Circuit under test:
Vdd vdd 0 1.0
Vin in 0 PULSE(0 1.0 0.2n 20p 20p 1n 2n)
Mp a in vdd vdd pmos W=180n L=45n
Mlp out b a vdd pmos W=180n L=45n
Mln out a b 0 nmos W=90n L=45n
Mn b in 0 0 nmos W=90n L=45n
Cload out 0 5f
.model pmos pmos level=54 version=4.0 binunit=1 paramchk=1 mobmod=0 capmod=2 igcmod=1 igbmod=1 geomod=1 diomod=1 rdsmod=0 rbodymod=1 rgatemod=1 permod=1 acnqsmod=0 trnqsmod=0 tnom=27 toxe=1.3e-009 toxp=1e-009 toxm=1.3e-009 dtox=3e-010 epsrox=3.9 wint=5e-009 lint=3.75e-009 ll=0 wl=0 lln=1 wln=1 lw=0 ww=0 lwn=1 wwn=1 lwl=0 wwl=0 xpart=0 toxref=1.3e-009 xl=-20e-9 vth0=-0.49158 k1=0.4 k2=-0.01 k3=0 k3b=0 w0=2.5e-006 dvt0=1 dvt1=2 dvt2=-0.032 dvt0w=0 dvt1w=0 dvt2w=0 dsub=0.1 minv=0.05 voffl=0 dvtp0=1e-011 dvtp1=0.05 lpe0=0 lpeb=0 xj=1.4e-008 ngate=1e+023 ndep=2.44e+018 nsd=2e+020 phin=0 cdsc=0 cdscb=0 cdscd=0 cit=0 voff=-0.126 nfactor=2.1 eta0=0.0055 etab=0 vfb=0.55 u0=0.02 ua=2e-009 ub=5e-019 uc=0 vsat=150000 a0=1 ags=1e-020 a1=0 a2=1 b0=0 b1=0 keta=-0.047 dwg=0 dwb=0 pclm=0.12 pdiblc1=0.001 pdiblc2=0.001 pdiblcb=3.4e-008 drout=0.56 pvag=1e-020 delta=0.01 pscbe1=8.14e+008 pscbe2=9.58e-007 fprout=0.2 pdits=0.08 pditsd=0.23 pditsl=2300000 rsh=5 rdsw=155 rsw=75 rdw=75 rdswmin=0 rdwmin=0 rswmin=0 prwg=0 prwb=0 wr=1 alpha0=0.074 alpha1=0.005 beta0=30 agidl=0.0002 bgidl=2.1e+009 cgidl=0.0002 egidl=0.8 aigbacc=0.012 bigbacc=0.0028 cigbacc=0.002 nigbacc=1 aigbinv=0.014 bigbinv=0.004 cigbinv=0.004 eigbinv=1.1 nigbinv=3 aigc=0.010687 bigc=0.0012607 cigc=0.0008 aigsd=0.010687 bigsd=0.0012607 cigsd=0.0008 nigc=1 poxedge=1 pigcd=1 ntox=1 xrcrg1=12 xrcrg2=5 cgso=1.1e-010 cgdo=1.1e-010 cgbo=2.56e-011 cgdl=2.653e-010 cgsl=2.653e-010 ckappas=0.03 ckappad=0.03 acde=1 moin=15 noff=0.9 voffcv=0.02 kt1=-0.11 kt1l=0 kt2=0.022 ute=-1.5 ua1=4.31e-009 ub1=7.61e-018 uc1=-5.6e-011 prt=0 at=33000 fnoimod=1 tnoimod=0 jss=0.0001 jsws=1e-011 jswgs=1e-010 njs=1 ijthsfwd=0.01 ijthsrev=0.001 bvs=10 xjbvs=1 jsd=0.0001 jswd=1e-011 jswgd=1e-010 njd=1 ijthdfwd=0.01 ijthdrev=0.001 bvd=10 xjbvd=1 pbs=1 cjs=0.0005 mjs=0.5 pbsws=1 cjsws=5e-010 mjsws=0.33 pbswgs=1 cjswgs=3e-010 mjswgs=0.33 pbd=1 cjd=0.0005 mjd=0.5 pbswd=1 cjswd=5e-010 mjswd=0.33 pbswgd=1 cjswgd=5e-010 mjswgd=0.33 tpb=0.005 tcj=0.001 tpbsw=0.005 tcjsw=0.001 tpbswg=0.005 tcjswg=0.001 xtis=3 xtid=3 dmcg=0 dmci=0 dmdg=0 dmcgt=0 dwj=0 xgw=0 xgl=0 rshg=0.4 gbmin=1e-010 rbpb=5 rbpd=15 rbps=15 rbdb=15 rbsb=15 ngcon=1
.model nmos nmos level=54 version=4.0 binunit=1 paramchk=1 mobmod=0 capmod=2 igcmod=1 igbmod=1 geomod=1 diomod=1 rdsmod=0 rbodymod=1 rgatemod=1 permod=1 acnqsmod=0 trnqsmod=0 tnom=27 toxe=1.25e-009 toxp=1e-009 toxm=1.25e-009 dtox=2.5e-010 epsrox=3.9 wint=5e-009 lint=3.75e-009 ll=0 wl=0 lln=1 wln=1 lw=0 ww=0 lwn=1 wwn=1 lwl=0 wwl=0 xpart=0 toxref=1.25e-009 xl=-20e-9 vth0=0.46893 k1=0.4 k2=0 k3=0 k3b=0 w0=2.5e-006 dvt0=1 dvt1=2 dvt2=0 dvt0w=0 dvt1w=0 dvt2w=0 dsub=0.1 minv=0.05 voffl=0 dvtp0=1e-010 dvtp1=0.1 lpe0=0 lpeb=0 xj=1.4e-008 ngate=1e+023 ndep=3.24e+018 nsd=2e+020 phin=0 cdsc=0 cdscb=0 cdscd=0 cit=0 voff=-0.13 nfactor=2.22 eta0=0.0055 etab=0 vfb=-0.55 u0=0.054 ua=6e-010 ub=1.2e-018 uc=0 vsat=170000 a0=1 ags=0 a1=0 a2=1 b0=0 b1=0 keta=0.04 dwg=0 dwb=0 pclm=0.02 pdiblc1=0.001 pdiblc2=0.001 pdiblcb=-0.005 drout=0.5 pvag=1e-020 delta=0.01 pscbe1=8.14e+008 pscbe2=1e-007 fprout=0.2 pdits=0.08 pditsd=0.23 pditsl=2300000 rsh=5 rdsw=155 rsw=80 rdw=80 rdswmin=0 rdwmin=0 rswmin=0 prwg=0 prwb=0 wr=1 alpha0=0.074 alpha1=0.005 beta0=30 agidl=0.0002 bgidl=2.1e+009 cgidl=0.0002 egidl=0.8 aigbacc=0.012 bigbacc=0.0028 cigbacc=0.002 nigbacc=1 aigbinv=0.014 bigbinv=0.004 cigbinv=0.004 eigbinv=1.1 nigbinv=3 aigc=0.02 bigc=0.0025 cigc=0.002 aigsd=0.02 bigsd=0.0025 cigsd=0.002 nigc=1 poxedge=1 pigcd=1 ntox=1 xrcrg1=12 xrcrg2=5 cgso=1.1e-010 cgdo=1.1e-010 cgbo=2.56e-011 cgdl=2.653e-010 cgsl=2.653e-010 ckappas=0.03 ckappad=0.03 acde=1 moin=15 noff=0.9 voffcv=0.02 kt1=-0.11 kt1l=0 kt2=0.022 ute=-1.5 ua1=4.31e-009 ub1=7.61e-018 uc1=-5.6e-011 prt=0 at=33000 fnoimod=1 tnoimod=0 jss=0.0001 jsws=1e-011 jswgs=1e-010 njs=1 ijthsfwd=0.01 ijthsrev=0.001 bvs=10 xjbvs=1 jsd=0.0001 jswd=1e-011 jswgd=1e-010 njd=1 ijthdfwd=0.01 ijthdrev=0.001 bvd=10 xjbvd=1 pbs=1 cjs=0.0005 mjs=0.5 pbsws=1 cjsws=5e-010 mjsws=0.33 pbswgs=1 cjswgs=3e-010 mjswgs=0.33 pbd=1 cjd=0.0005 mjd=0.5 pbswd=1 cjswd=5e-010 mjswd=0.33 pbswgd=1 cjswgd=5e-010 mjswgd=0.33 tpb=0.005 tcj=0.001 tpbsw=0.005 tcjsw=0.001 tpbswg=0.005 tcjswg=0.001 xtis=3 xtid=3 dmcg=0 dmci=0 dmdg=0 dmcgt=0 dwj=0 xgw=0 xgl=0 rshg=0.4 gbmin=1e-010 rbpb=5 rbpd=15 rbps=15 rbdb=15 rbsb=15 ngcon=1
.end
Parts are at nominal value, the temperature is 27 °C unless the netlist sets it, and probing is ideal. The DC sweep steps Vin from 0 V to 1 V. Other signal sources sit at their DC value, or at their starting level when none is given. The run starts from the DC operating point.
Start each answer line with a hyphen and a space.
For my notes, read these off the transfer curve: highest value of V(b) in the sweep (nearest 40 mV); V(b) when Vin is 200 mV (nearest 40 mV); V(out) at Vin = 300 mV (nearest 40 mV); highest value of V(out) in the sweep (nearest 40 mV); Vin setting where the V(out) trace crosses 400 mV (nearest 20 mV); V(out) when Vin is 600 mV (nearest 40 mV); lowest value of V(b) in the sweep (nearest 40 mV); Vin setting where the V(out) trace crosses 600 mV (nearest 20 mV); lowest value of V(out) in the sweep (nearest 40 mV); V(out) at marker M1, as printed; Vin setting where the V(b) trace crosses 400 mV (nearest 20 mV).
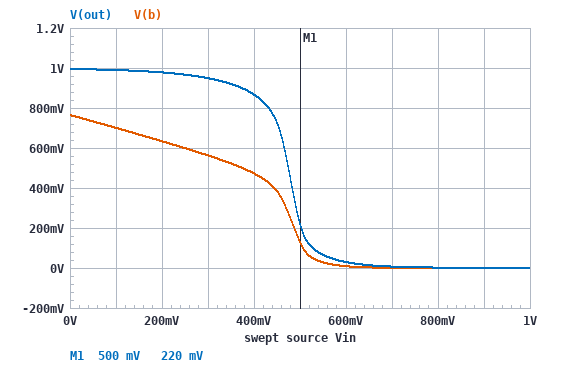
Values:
- 760 mV
- 640 mV
- 960 mV
- 1.00 V
- 480 mV
- 40 mV
- 0 V
- 460 mV
- 0 V
- 220 mV
- 440 mV
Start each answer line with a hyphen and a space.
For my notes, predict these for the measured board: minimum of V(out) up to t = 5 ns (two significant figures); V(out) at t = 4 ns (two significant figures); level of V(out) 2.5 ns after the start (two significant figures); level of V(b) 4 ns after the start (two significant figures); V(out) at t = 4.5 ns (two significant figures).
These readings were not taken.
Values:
- 120 mV
- 680 mV
- 260 mV
- 640 mV
- 260 mV
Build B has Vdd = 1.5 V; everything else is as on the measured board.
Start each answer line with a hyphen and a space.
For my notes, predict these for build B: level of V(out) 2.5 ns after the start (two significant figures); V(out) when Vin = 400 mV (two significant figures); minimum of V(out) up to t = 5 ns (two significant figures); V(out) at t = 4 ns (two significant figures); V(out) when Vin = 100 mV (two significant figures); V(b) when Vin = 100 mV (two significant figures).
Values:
- 160 mV
- 1.4 V
- 140 mV
- 1.3 V
- 1.5 V
- 1.1 V
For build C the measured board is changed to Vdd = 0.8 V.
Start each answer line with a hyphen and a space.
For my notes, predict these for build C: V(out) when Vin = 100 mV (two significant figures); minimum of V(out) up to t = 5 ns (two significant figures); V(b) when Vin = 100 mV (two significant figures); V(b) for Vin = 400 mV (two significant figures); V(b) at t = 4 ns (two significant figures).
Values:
- 780 mV
- 170 mV
- 540 mV
- 57 mV
- 450 mV
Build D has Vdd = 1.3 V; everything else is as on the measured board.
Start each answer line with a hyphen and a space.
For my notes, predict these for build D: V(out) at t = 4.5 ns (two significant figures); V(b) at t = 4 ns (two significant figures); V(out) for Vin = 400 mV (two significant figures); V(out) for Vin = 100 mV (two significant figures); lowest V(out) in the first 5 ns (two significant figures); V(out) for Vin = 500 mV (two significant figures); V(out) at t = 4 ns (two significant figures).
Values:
- 130 mV
- 920 mV
- 1.2 V
- 1.3 V
- 8.5 mV
- 1.1 V
- 1.0 V
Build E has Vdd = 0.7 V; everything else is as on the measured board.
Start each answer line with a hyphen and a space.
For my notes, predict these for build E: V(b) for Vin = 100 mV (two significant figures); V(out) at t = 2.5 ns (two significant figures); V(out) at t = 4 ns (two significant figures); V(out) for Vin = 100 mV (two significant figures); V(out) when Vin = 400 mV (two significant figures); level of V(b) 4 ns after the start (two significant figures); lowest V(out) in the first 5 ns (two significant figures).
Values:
- 460 mV
- 240 mV
- 360 mV
- 670 mV
- 12 mV
- 350 mV
- 170 mV
